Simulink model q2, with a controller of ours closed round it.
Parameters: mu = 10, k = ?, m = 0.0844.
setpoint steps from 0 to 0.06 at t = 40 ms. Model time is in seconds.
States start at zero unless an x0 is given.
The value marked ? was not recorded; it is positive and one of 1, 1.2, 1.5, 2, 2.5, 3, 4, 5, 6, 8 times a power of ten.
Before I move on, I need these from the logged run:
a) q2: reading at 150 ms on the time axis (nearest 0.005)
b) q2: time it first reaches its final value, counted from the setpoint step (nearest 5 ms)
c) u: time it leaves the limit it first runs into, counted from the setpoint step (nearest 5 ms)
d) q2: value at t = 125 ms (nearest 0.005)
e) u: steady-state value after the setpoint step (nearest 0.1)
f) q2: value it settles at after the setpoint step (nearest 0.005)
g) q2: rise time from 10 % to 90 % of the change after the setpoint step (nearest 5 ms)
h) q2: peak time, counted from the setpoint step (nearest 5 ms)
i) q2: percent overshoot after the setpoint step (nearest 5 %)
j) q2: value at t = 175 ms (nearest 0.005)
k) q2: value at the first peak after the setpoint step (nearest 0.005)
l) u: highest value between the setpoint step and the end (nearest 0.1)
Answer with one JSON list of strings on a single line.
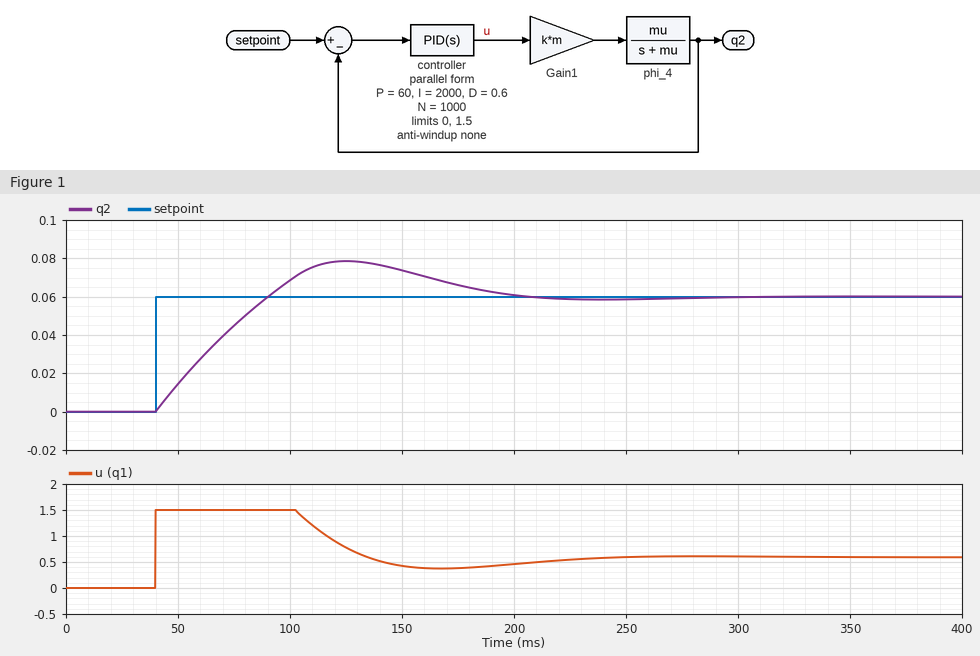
["0.075", "50 ms", "65 ms", "0.080", "0.6", "0.060", "40 ms", "85 ms", "30 %", "0.065", "0.080", "1.5"]
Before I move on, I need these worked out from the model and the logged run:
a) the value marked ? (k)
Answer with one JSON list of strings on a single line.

["1.2"]
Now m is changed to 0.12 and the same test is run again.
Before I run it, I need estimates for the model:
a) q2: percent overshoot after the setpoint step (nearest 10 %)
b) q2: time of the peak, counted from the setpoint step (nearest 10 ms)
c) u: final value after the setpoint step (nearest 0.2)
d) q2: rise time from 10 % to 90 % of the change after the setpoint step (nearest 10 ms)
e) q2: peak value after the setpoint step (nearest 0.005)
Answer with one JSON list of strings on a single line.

["20 %", "60 ms", "0.4", "30 ms", "0.075"]
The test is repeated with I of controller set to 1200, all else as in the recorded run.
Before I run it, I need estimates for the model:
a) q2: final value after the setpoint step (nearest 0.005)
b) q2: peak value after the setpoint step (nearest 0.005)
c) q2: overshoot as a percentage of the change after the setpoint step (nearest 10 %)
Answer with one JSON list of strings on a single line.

["0.060", "0.070", "20 %"]
